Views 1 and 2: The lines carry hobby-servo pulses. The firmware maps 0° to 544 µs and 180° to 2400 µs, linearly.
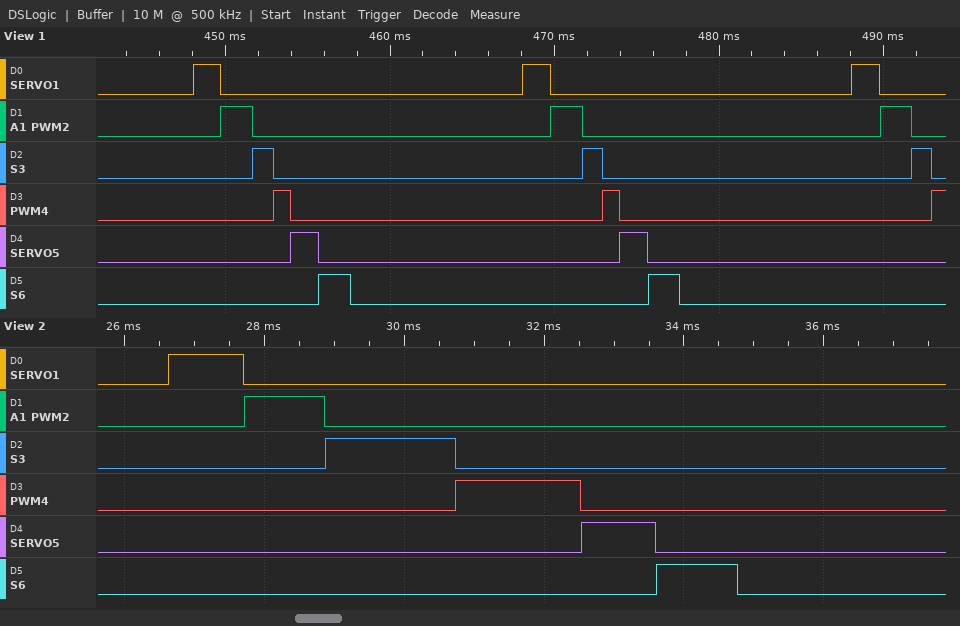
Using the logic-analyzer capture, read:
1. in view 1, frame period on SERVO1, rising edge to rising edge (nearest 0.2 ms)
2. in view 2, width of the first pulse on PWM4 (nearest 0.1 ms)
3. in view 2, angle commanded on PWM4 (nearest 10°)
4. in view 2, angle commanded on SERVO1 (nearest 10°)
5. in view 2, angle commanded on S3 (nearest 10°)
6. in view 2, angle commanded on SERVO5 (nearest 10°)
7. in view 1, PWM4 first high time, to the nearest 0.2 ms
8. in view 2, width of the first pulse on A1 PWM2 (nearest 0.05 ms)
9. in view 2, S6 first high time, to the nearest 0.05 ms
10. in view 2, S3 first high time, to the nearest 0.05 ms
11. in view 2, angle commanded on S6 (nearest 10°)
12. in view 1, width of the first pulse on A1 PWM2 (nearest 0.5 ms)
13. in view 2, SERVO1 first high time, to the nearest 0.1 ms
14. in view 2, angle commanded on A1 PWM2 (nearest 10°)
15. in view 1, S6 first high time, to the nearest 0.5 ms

20.0 ms
1.8 ms
120°
50°
130°
50°
1.0 ms
1.15 ms
1.15 ms
1.85 ms
60°
2.0 ms
1.1 ms
60°
2.0 ms
